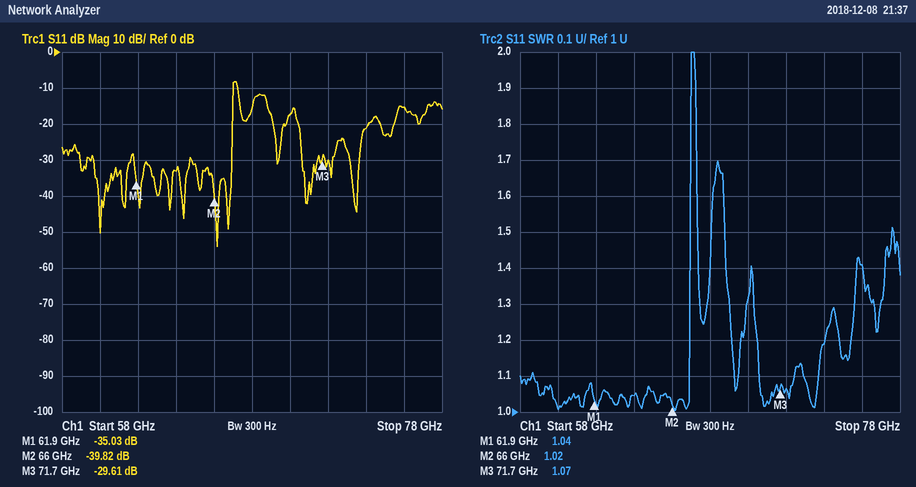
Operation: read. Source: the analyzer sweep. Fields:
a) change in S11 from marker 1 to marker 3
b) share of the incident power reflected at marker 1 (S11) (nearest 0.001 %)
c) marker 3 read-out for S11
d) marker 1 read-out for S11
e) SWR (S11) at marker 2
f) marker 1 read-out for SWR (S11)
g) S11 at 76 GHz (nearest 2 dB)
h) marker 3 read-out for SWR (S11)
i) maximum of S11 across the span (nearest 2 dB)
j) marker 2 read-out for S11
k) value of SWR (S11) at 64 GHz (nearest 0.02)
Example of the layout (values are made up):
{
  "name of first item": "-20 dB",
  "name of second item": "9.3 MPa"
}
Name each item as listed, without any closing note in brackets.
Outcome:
{
  "change in S11 from marker 1 to marker 3": "5.42 dB",
  "share of the incident power reflected at marker 1 (S11)": "0.031 %",
  "marker 3 read-out for S11": "-29.61 dB",
  "marker 1 read-out for S11": "-35.03 dB",
  "SWR (S11) at marker 2": "1.02",
  "marker 1 read-out for SWR": "1.04",
  "S11 at 76 GHz": "-16 dB",
  "marker 3 read-out for SWR": "1.07",
  "maximum of S11 across the span": "-8 dB",
  "marker 2 read-out for S11": "-39.82 dB",
  "value of SWR (S11) at 64 GHz": "1.04"
}
